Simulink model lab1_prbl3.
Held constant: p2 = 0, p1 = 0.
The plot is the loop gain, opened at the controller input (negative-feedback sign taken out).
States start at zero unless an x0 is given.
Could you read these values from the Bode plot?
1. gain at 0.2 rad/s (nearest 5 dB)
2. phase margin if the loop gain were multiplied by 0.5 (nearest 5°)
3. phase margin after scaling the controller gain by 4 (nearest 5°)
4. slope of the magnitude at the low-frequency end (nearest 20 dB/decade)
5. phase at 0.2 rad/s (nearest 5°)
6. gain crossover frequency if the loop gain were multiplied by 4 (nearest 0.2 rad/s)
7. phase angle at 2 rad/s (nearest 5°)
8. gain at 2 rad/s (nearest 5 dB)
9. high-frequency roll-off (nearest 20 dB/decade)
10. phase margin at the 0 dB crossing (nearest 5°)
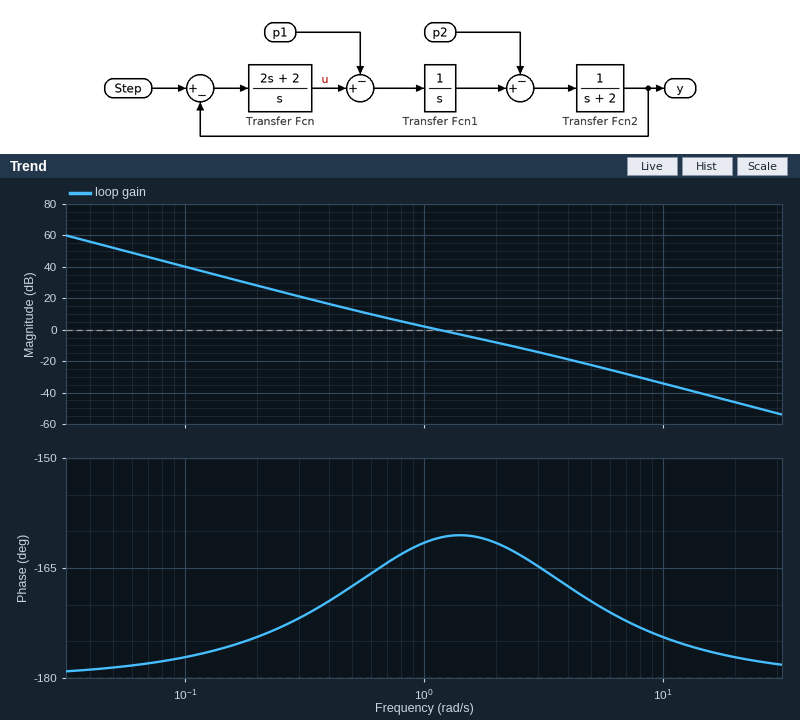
30 dB
15°
15°
-40 dB/decade
-175°
2.6 rad/s
-160°
-10 dB
-40 dB/decade
20°
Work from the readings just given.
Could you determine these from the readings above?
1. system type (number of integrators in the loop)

2
